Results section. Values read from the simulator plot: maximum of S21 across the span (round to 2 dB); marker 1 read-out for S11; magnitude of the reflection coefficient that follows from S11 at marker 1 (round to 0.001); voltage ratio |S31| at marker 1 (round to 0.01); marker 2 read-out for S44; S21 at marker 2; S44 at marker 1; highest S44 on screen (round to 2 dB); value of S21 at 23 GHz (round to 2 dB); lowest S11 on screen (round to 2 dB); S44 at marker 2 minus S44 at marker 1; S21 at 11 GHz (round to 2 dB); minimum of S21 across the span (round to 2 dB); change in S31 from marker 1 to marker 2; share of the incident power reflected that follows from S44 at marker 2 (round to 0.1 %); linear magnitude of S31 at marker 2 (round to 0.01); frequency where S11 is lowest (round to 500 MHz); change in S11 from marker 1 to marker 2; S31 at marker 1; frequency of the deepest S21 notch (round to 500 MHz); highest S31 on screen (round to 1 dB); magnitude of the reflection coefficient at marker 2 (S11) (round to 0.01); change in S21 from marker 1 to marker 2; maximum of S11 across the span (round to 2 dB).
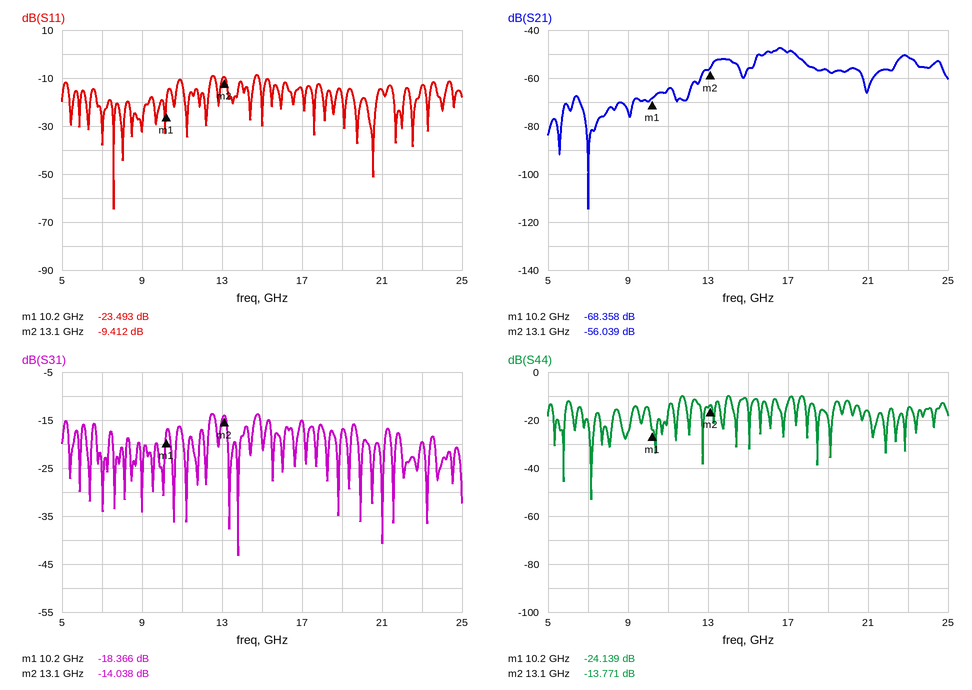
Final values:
-48 dB
-23.493 dB
0.067
0.12
-13.771 dB
-56.039 dB
-24.139 dB
-10 dB
-52 dB
-64 dB
10.368 dB
-64 dB
-114 dB
4.328 dB
4.2 %
0.20
7.5 GHz
14.081 dB
-18.366 dB
7.0 GHz
-14 dB
0.34
12.319 dB
-8 dB
